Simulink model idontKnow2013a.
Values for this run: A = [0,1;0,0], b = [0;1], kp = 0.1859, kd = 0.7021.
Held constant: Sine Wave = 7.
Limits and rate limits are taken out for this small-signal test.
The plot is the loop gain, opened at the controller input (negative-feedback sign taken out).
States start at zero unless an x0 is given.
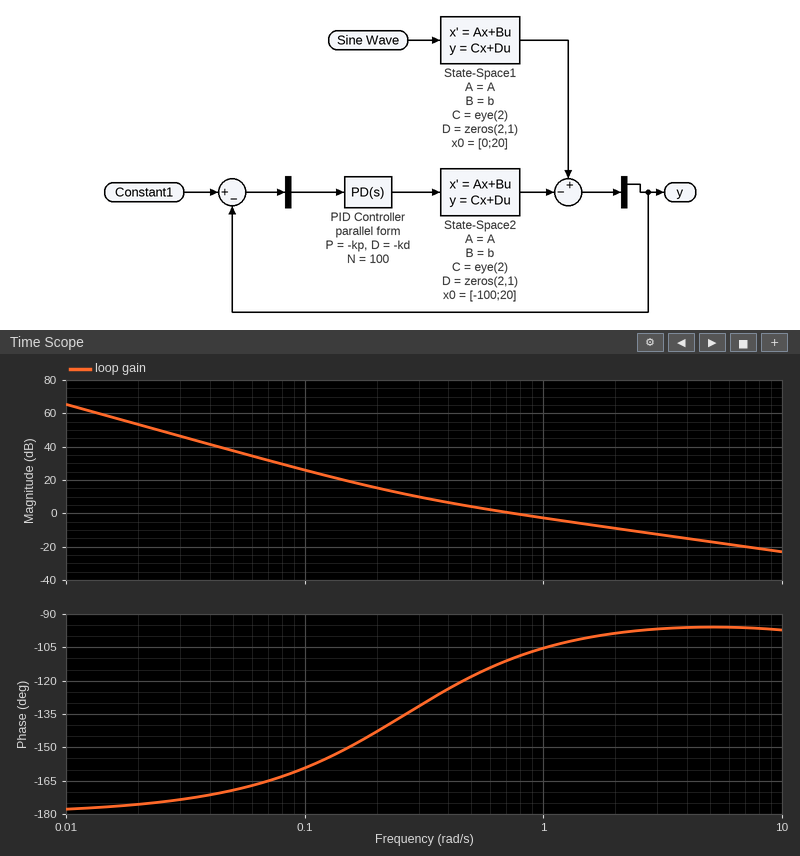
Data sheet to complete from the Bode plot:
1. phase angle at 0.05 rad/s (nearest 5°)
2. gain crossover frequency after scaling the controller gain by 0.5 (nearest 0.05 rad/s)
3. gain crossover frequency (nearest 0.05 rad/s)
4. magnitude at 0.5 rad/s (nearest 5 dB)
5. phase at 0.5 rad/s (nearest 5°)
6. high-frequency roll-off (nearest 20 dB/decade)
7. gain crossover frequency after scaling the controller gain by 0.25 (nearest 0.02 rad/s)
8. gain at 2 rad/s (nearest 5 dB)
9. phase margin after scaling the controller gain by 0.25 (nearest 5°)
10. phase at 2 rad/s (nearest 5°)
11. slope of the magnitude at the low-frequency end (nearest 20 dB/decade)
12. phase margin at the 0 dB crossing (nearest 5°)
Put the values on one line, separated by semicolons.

-170°; 0.40 rad/s; 0.75 rad/s; 5 dB; -120°; -20 dB/decade; 0.26 rad/s; -10 dB; 45°; -100°; -40 dB/decade; 70°
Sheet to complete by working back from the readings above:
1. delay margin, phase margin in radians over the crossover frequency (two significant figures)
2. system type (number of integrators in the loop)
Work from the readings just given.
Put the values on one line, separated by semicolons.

1.6 s; 2
